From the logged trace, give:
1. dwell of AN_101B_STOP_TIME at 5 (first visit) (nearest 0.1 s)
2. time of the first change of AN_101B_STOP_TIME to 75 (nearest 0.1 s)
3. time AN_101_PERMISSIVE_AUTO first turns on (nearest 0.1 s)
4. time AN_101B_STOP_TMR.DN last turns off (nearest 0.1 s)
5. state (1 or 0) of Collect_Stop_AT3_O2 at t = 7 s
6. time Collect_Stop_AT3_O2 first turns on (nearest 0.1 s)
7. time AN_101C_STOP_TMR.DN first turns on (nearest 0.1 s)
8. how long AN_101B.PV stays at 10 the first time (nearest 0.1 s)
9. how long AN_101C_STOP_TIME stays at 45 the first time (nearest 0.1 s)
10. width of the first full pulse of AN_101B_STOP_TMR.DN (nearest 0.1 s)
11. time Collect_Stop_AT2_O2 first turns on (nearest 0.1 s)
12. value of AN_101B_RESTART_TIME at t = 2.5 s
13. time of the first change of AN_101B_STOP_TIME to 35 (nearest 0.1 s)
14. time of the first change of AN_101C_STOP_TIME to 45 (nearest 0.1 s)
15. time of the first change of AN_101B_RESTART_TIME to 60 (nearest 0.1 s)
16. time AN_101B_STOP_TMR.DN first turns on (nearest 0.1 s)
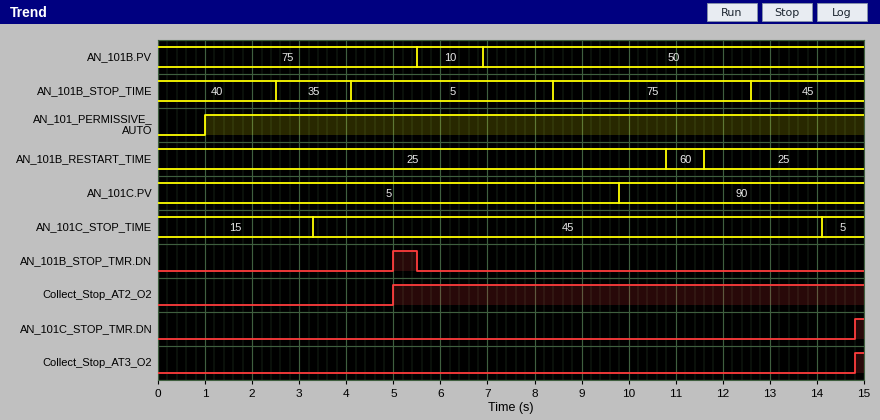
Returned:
4.3 s
8.4 s
1.0 s
5.5 s
0
14.8 s
14.8 s
1.4 s
10.8 s
0.5 s
5.0 s
25
2.5 s
3.3 s
10.8 s
5.0 s
